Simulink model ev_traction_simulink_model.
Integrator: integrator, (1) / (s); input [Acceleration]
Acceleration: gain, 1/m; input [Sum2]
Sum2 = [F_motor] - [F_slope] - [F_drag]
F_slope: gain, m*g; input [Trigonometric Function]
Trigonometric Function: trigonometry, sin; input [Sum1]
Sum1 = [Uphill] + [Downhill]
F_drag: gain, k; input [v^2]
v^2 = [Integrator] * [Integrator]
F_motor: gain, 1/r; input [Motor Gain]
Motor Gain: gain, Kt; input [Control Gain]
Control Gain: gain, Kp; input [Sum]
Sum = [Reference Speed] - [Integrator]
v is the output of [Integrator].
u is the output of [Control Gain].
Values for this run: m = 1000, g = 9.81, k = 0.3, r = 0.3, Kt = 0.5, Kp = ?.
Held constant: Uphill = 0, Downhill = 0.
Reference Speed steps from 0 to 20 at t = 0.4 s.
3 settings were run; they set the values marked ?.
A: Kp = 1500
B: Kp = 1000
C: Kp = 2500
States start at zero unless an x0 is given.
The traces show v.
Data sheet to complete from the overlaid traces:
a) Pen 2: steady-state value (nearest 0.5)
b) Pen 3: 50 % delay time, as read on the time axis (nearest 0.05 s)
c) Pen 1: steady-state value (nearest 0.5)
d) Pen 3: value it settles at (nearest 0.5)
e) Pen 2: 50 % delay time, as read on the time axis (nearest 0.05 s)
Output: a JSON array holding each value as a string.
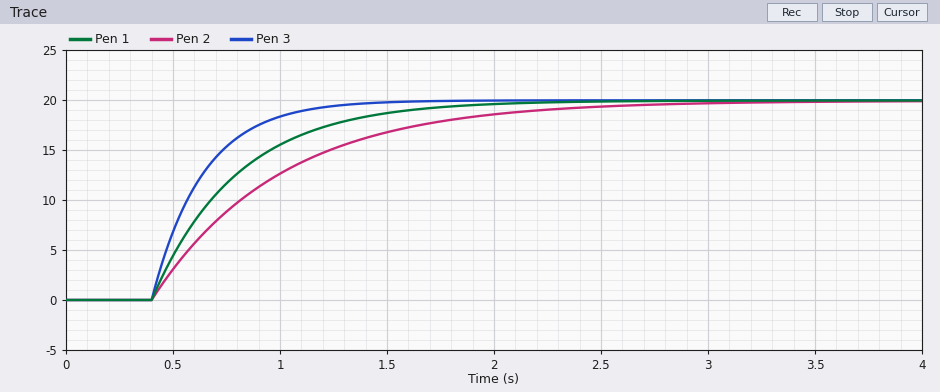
["20.0", "0.55 s", "20.0", "20.0", "0.80 s"]
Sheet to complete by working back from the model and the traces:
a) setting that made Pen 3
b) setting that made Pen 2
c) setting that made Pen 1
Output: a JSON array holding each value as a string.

["C", "B", "A"]
